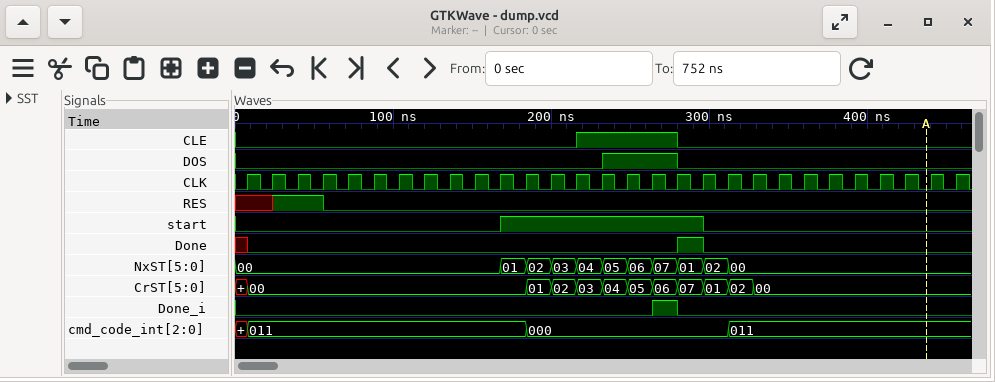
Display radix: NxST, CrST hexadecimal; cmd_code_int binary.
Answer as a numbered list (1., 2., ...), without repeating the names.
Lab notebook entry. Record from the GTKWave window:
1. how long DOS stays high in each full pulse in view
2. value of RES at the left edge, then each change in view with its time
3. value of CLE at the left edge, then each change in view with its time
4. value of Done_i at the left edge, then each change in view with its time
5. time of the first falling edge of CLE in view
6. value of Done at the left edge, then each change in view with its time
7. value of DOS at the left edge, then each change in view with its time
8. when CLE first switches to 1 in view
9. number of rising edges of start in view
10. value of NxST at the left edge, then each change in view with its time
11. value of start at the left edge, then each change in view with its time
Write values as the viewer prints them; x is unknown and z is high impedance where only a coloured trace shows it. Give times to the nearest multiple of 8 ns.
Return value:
1. 48 ns
2. x, 1 at 24 ns, 0 at 56 ns
3. 0, 1 at 216 ns, 0 at 280 ns
4. 0, 1 at 264 ns, 0 at 280 ns
5. 280 ns
6. x, 0 at 8 ns, 1 at 280 ns, 0 at 296 ns
7. 0, 1 at 232 ns, 0 at 280 ns
8. 216 ns
9. 1
10. 00, 01 at 168 ns, 02 at 184 ns, 03 at 200 ns, 04 at 216 ns, 05 at 232 ns, 06 at 248 ns, 07 at 264 ns, 01 at 280 ns, 02 at 296 ns, 00 at 312 ns
11. 0, 1 at 168 ns, 0 at 296 ns
